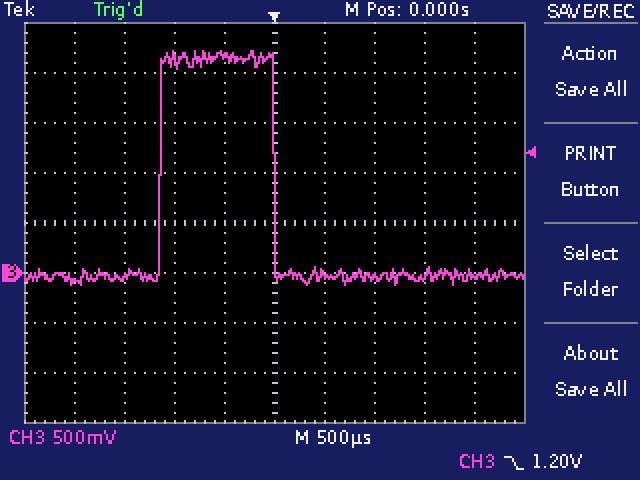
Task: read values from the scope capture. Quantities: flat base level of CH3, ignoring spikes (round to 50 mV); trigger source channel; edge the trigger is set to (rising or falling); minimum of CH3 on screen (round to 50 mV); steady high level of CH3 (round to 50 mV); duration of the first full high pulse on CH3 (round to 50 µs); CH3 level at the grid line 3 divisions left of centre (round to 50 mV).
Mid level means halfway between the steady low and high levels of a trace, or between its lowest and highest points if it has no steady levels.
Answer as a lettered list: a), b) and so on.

a) -50 mV
b) CH3
c) falling
d) -100 mV
e) 2.15 V
f) 1.15 ms
g) -50 mV
